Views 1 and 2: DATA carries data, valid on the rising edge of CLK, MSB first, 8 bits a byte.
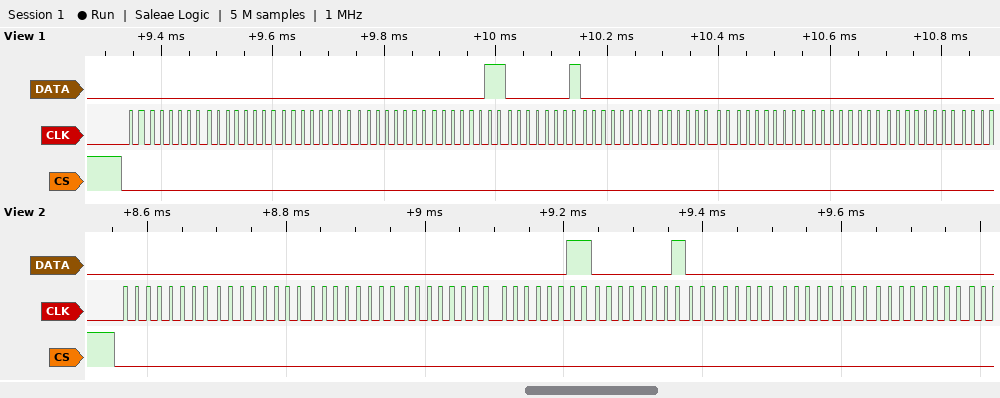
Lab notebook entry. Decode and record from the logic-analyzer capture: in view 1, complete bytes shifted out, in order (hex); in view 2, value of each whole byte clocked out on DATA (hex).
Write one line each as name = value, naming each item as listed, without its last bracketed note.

in view 1, complete bytes shifted out, in order = 00 00 00 00 03 01 00 00 00 00 00
in view 2, value of each whole byte clocked out on DATA = 00 00 00 00 03 01 00 00 00
